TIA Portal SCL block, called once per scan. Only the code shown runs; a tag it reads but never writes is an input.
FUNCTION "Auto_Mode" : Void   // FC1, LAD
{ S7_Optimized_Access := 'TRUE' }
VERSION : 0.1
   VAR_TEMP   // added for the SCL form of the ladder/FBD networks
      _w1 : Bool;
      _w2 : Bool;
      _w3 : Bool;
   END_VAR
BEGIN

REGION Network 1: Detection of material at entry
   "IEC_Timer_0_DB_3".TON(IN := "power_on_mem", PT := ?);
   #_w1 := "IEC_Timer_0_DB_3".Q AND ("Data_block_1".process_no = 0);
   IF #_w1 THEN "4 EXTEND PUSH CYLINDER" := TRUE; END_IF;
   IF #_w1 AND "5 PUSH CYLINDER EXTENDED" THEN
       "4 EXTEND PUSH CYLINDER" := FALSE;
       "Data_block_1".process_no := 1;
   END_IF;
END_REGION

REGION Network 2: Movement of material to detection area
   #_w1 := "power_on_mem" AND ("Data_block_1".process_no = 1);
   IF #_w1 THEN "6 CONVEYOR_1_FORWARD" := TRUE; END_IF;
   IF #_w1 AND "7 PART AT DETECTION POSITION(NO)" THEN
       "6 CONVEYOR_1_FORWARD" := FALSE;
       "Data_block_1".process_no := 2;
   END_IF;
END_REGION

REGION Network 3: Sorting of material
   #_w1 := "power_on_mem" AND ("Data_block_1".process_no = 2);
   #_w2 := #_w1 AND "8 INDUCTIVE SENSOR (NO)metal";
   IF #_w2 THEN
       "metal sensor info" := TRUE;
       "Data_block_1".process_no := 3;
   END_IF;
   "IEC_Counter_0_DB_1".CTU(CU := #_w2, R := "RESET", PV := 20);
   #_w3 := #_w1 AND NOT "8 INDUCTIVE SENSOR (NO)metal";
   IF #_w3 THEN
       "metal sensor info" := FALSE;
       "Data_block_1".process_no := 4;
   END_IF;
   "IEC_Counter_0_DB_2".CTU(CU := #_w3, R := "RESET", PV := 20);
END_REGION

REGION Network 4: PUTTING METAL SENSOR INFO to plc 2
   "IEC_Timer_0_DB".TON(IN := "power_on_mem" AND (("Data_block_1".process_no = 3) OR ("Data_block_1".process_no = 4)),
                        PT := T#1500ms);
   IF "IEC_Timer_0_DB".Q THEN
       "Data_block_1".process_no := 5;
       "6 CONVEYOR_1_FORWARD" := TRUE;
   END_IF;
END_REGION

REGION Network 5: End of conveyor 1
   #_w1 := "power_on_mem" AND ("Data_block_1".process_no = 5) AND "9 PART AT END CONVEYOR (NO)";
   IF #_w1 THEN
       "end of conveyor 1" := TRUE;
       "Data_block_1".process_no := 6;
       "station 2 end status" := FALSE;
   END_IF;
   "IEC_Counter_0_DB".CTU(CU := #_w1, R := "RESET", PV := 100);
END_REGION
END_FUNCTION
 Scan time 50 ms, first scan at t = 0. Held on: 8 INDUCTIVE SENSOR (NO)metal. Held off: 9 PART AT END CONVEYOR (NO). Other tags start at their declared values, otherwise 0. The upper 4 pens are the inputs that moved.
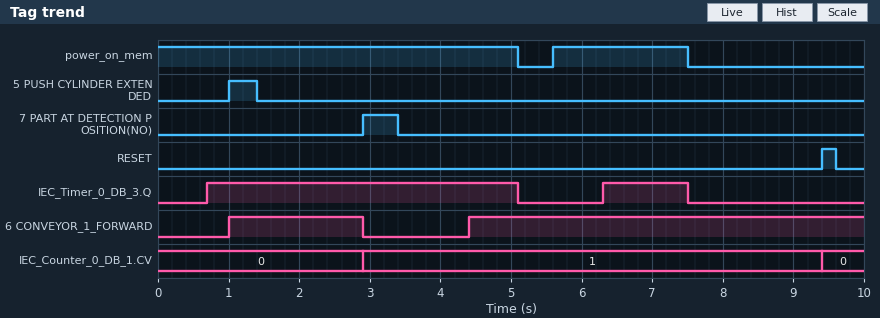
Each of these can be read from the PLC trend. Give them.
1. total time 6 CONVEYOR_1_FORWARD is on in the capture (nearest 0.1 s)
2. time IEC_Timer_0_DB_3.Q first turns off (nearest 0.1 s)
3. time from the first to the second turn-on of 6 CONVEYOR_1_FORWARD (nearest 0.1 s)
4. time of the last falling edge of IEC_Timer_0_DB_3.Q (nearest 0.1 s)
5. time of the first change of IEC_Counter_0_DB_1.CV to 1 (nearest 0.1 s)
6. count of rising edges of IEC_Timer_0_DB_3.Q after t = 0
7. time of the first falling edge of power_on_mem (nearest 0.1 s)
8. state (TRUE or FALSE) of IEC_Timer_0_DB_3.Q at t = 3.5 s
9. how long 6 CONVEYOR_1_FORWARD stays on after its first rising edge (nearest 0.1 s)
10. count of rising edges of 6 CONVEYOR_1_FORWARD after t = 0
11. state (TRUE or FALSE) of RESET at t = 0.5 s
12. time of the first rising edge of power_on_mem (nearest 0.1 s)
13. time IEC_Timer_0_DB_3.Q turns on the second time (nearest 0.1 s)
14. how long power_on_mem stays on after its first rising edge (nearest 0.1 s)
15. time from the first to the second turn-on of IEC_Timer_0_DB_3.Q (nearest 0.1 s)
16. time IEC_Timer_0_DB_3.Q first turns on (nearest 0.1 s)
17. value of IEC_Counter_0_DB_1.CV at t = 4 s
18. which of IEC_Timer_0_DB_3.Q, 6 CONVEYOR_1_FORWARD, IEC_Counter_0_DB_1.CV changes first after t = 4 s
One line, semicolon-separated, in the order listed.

7.5 s; 5.1 s; 3.4 s; 7.5 s; 2.9 s; 2; 5.1 s; TRUE; 1.9 s; 2; FALSE; 5.6 s; 6.3 s; 1.9 s; 5.6 s; 0.7 s; 1; 6 CONVEYOR_1_FORWARD
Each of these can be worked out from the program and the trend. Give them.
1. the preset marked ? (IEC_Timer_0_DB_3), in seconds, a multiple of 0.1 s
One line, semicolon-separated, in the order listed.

0.7 s
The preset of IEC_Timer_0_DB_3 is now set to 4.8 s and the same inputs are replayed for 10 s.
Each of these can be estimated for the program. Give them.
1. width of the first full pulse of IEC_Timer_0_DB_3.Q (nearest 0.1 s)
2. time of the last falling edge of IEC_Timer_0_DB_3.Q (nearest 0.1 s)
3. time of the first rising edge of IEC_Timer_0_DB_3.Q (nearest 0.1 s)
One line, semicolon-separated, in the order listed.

0.3 s; 5.1 s; 4.8 s
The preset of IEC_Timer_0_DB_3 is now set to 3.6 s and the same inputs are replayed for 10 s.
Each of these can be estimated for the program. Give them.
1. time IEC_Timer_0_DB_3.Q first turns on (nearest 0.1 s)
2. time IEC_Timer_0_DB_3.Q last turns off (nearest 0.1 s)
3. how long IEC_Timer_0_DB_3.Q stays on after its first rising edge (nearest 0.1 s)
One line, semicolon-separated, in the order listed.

3.6 s; 5.1 s; 1.5 s
